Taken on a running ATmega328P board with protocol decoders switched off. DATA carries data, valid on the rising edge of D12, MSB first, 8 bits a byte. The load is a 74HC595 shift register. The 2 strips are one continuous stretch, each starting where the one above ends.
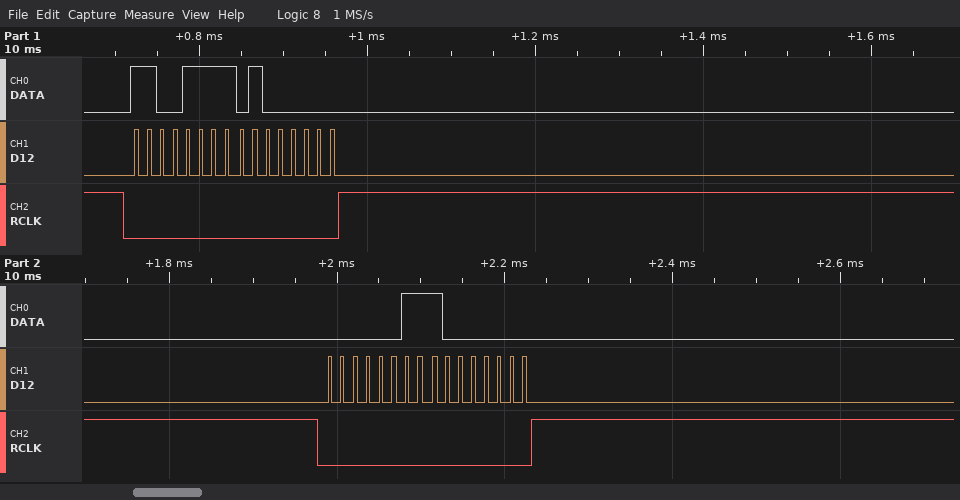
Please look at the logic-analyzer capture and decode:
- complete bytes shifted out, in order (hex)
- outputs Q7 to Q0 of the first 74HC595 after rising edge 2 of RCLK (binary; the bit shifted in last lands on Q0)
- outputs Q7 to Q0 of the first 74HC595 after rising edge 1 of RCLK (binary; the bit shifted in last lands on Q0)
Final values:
0xCF 0x40 0x03 0x80
10000000
01000000
